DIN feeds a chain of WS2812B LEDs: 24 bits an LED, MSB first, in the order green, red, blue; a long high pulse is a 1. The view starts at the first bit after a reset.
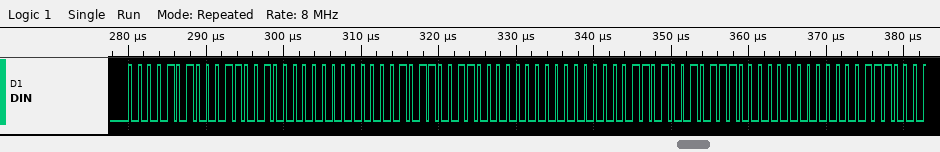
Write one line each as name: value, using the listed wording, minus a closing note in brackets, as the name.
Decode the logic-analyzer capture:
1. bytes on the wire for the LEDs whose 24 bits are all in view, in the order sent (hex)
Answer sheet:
bytes on the wire for the LEDs whose 24 bits are all in view, in the order sent: 0A 32 00 0B 30 00 0D 2E 00
